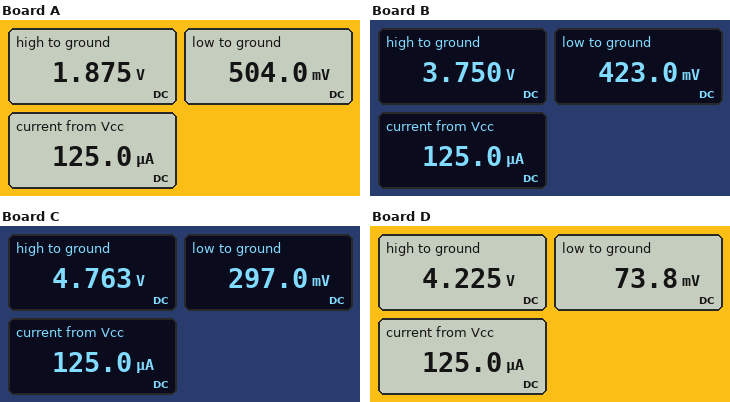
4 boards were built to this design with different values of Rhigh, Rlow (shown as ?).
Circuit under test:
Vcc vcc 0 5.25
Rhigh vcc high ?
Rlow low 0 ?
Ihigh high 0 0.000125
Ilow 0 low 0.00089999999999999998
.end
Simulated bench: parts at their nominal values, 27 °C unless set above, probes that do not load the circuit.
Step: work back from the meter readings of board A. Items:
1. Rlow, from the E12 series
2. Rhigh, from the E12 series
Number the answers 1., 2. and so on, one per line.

1. 560 Ω
2. 27 kΩ
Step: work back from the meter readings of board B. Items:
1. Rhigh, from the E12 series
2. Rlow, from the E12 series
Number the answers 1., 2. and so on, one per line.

1. 12 kΩ
2. 470 Ω
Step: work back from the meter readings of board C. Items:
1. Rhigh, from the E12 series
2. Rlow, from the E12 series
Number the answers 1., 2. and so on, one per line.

1. 3.9 kΩ
2. 330 Ω
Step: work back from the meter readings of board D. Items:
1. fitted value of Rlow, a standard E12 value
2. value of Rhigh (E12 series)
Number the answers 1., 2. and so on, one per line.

1. 82 Ω
2. 8.2 kΩ
